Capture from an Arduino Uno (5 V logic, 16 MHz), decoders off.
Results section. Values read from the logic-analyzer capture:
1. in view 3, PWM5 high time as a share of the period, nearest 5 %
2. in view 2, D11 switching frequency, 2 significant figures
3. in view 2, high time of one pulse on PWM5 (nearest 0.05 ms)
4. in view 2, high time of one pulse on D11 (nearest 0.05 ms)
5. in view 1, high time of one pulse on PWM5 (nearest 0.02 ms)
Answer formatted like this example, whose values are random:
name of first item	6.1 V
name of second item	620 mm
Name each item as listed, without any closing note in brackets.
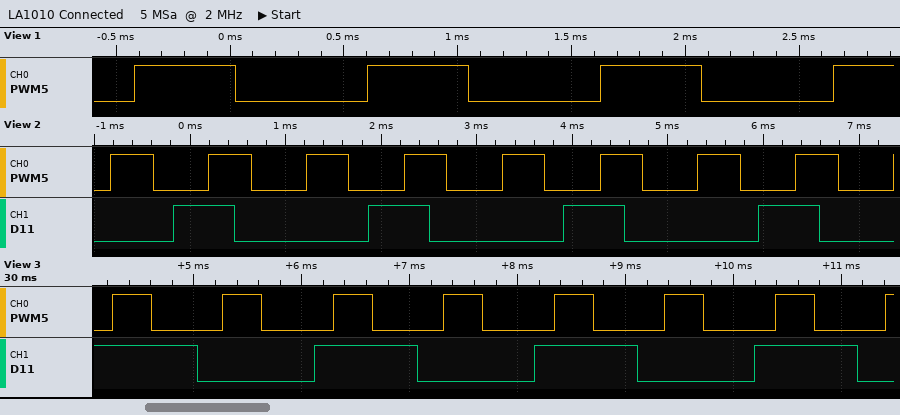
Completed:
in view 3, PWM5 high time as a share of the period, nearest 5 %	35 %
in view 2, D11 switching frequency, 2 significant figures	490 Hz
in view 2, high time of one pulse on PWM5	0.45 ms
in view 2, high time of one pulse on D11	0.65 ms
in view 1, high time of one pulse on PWM5	0.44 ms
